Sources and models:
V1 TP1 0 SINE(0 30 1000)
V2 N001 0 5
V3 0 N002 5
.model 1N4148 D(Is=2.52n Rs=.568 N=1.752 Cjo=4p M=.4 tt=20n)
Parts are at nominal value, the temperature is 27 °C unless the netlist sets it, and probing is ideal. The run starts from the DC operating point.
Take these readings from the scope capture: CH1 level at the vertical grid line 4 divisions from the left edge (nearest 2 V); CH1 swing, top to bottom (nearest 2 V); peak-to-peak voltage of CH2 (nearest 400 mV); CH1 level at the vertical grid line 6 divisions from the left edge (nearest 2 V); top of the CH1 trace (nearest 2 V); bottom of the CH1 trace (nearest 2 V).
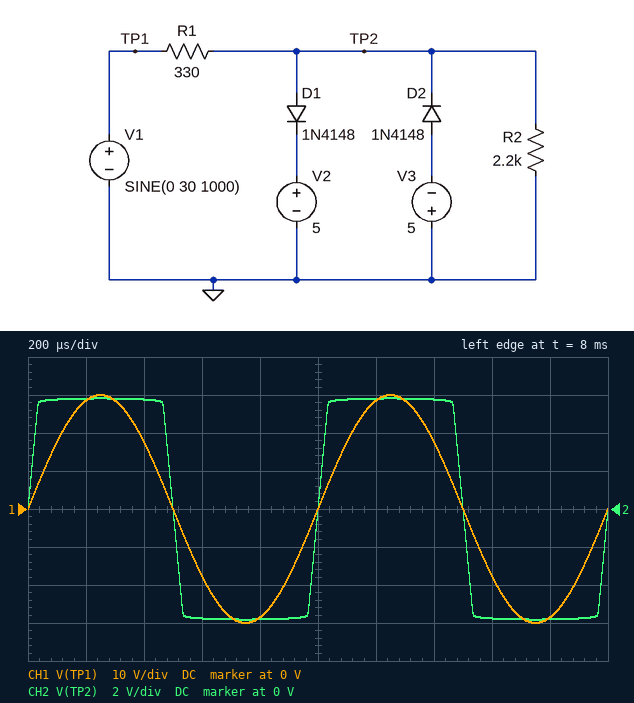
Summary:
-28 V
60 V
11.6 V
28 V
30 V
-30 V
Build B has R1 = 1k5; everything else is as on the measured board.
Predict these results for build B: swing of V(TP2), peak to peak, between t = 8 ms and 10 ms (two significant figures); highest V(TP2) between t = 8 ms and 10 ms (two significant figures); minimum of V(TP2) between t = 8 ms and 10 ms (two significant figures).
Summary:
11 V
5.7 V
-5.7 V
